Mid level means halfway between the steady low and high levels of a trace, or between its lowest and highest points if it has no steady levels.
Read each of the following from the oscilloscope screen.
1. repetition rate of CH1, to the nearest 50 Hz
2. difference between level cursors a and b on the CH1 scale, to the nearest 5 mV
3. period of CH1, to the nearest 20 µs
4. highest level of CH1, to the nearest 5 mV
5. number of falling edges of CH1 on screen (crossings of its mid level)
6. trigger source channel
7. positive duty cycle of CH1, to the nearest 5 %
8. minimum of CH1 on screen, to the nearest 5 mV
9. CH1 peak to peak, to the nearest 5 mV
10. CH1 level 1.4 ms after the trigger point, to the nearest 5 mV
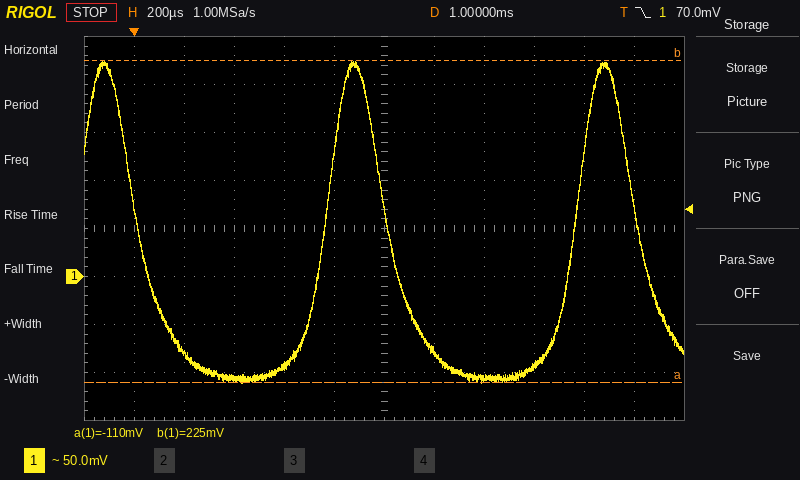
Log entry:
1.00 kHz
335 mV
1.00 ms
225 mV
3
CH1
25 %
-110 mV
335 mV
-105 mV
